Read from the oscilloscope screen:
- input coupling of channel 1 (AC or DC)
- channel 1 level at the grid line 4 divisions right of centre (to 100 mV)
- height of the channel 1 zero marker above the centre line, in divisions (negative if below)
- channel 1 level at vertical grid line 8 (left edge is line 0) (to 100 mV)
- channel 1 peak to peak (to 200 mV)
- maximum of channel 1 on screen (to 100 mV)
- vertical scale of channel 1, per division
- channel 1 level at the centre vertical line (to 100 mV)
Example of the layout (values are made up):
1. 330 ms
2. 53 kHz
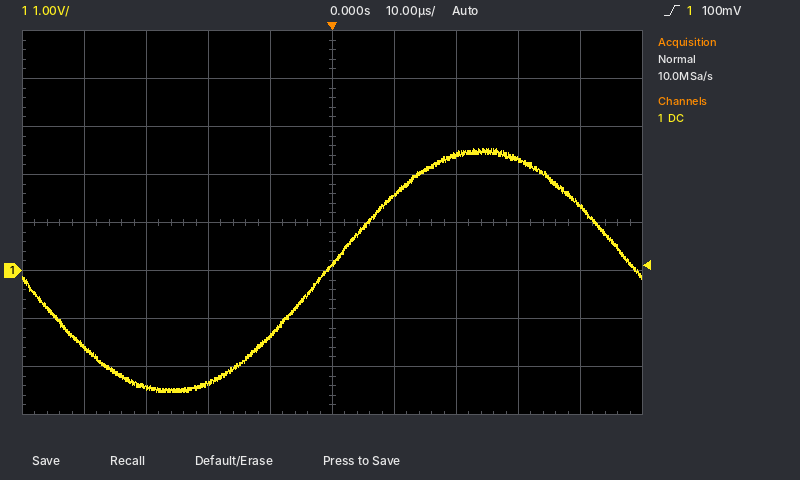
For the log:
1. DC
2. 1.3 V
3. -1.0 div
4. 2.3 V
5. 5.0 V
6. 2.5 V
7. 1 V
8. 100 mV
